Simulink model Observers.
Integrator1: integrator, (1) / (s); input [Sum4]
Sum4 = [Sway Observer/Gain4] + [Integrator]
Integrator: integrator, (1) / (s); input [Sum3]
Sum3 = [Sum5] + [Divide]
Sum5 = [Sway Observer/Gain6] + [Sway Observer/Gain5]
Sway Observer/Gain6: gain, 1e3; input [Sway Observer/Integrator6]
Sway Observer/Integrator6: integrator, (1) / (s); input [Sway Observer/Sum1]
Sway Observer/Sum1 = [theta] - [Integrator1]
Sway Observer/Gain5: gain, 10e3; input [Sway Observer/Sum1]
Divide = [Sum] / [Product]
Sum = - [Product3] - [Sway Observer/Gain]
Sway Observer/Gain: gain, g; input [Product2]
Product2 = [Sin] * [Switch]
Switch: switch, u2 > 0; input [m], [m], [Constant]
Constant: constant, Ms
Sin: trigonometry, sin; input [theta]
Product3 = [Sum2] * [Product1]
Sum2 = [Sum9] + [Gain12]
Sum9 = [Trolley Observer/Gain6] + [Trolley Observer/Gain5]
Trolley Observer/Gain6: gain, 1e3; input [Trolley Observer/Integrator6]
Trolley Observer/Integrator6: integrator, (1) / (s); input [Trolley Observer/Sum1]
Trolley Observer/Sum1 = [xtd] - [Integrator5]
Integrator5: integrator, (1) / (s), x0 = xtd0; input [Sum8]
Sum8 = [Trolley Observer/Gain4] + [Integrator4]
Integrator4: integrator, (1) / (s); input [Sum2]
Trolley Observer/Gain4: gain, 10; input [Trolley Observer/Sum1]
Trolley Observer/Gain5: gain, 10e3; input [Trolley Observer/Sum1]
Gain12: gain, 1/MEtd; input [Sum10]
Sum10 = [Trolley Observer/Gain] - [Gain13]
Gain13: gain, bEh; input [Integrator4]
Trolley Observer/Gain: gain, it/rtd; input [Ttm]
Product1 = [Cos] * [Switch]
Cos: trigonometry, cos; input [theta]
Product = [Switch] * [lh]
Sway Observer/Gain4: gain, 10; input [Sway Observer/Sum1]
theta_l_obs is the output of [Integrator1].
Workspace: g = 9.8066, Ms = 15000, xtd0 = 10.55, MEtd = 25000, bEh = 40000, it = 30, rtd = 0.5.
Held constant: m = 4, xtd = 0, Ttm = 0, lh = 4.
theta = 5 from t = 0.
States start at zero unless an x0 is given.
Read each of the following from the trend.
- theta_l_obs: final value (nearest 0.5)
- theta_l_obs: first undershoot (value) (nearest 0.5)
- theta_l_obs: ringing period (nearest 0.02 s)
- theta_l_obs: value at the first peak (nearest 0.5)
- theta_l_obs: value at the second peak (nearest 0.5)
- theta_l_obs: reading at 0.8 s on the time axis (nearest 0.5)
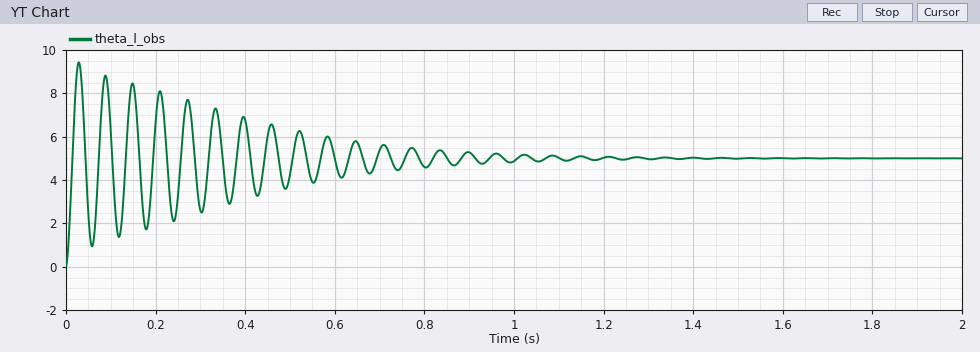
5.0
1.0
0.06 s
9.5
9.0
4.5
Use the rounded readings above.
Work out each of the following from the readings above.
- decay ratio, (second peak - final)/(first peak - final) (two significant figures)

0.89
